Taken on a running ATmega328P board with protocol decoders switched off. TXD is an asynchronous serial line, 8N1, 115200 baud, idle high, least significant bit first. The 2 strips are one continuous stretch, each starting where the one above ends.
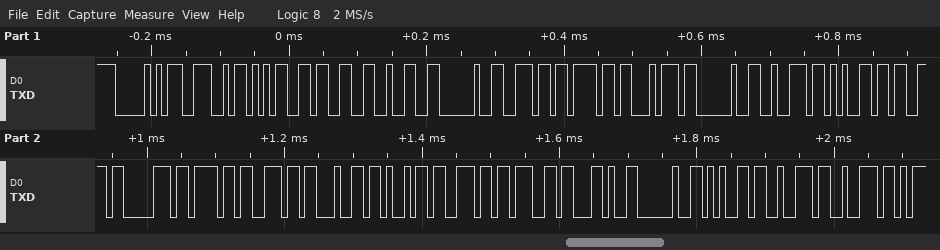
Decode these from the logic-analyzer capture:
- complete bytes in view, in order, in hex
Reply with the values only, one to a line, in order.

0x50 0x4E 0x35 0x33 0x32 0x20 0x6E 0x6F 0x74 0x20 0x72 0x65 0x73 0x70 0x6F 0x6E 0x64 0x69 0x6E 0x67 0x2C 0x20 0x65 0x72 0x72
